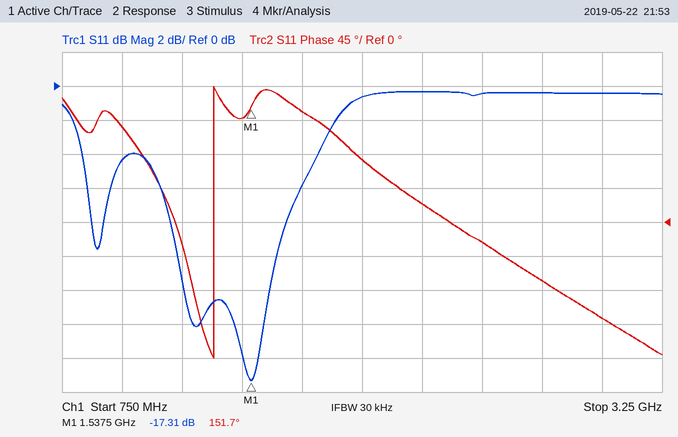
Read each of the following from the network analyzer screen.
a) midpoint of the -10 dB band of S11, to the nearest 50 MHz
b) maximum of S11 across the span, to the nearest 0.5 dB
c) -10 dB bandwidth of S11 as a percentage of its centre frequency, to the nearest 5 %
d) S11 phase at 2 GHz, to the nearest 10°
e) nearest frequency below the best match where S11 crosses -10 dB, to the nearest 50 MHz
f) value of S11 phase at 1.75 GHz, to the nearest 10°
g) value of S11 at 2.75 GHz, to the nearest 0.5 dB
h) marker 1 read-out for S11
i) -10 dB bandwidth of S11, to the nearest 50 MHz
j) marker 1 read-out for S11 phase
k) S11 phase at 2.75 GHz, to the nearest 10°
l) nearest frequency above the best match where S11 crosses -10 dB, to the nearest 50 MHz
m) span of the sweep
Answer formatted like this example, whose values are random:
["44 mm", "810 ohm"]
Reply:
["1.45 GHz", "-0.5 dB", "30 %", "80°", "1.25 GHz", "150°", "-0.5 dB", "-17.31 dB", "400 MHz", "151.7°", "-80°", "1.65 GHz", "2.5 GHz"]
